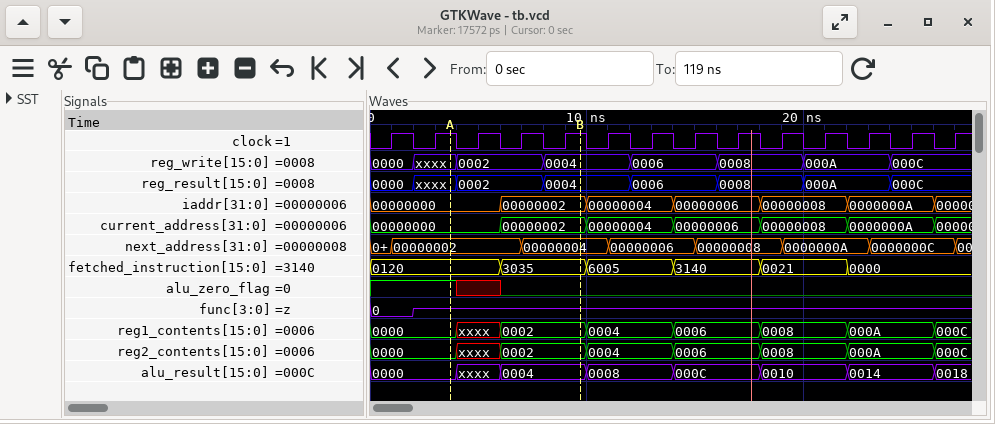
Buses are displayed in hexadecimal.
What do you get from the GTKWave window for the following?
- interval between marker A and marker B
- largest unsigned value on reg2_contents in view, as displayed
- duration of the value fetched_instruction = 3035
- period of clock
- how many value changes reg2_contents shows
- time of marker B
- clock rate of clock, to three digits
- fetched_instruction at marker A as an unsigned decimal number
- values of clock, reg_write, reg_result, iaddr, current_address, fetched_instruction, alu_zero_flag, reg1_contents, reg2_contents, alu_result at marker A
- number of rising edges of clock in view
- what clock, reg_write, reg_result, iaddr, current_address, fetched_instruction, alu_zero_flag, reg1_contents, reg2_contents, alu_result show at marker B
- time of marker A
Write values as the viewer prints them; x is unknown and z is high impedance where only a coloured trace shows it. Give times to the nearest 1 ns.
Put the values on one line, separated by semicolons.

6 ns; 000C; 4 ns; 2 ns; 7; 10 ns; 500 MHz; 288; clock=1, reg_write=xxxx, reg_result=xxxx, iaddr=00000000, current_address=00000000, fetched_instruction=0120, alu_zero_flag=1, reg1_contents=0000, reg2_contents=0000, alu_result=0000; 14; clock=1, reg_write=0004, reg_result=0004, iaddr=00000002, current_address=00000002, fetched_instruction=3035, alu_zero_flag=0, reg1_contents=0002, reg2_contents=0002, alu_result=0004; 4 ns
